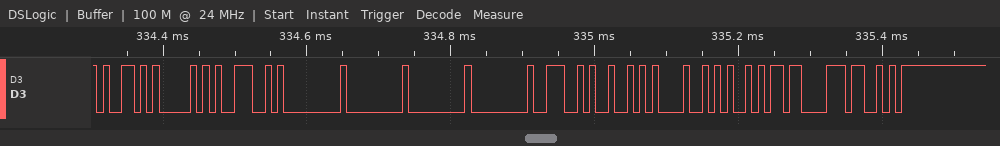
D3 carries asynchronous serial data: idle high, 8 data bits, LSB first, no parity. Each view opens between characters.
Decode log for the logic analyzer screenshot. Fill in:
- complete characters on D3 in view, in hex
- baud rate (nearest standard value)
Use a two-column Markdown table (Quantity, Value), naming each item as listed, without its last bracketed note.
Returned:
| Quantity | Value |
|---|---|
| complete characters on D3 in view, in hex | 59, 50, 4E, 00, 00, 00, 00, 4E, 52, 48, A9, C3, 53 |
| baud rate | 115200 baud |
